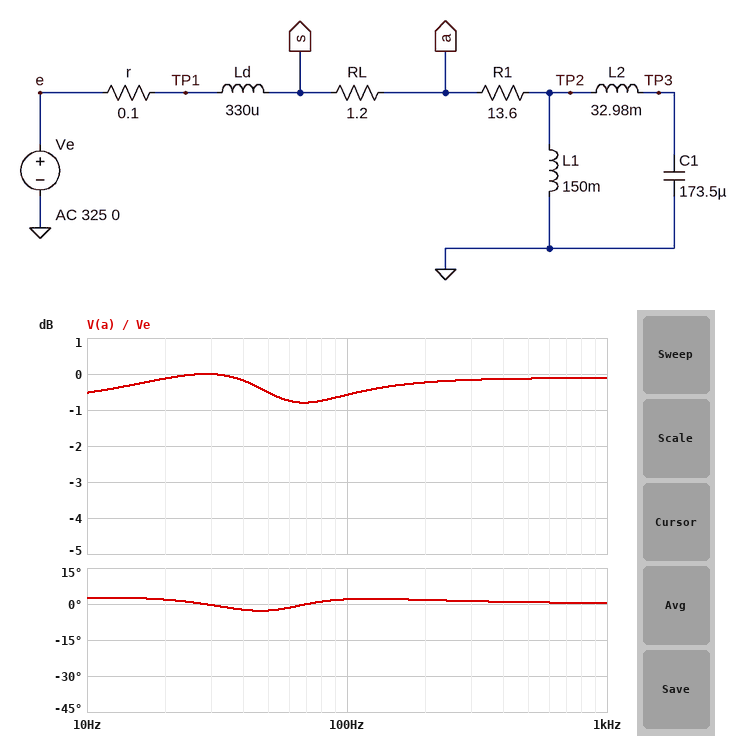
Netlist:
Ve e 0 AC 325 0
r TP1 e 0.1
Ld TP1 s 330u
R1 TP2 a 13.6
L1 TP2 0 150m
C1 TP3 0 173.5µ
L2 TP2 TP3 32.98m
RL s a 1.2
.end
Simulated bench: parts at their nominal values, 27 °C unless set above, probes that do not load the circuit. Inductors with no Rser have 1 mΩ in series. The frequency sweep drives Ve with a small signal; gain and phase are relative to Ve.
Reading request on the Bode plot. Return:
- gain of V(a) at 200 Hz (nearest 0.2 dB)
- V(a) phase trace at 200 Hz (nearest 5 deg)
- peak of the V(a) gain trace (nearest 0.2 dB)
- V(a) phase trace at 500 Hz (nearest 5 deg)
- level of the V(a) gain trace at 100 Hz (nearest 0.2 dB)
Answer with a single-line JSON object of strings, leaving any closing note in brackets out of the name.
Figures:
{"gain of V(a) at 200 Hz": "-0.2 dB", "V(a) phase trace at 200 Hz": "0 deg", "peak of the V(a) gain trace": "0 dB", "V(a) phase trace at 500 Hz": "0 deg", "level of the V(a) gain trace at 100 Hz": "-0.6 dB"}
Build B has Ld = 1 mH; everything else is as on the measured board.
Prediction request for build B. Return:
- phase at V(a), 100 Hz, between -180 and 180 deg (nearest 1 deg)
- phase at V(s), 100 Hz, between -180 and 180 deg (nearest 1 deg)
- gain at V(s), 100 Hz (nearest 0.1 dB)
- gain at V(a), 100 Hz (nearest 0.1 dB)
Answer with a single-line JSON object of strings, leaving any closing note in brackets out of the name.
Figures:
{"phase at V(a), 100 Hz, between -180 and 180 deg": "1 deg", "phase at V(s), 100 Hz, between -180 and 180 deg": "-1 deg", "gain at V(s), 100 Hz": "-0.2 dB", "gain at V(a), 100 Hz": "-0.7 dB"}
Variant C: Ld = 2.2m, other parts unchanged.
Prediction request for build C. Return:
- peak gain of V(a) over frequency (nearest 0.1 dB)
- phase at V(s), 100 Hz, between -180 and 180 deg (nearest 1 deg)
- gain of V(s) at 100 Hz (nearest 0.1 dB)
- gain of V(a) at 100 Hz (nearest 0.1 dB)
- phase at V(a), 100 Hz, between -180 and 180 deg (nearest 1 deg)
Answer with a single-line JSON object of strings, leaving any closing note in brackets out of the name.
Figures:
{"peak gain of V(a) over frequency": "0 dB", "phase at V(s), 100 Hz, between -180 and 180 deg": "-3 deg", "gain of V(s) at 100 Hz": "-0.4 dB", "gain of V(a) at 100 Hz": "-0.9 dB", "phase at V(a), 100 Hz, between -180 and 180 deg": "-1 deg"}
